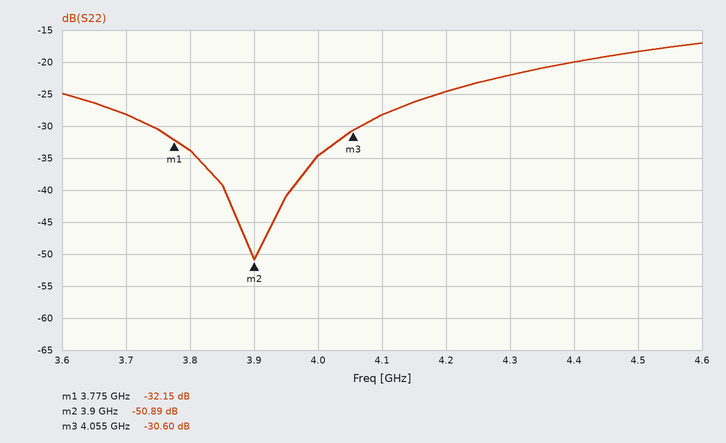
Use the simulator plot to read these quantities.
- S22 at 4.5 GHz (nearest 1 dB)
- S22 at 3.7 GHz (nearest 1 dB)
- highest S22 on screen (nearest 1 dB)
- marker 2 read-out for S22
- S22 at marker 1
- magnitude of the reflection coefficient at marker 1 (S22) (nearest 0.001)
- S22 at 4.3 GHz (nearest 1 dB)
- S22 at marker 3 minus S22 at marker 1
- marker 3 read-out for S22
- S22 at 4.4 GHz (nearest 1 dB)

-18 dB
-28 dB
-17 dB
-50.89 dB
-32.15 dB
0.025
-22 dB
1.55 dB
-30.60 dB
-20 dB
